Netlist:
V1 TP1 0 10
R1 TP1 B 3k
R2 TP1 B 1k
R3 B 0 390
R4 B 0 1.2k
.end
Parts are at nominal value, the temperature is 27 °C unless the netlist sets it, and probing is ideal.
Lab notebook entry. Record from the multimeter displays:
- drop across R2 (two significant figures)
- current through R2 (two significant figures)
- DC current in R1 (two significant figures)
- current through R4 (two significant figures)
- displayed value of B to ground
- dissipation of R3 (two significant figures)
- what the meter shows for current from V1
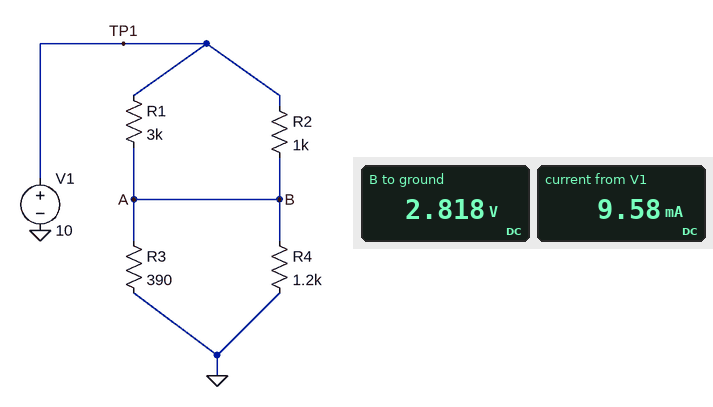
7.2 V
7.2 mA
2.4 mA
2.3 mA
2.818 V
20 mW
9.58 mA
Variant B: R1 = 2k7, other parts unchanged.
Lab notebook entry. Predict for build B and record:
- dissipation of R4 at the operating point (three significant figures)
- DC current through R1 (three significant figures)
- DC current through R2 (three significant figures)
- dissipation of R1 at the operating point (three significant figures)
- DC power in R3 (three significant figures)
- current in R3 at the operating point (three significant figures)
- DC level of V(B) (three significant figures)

6.88 mW
2.64 mA
7.13 mA
18.8 mW
21.2 mW
7.37 mA
2.87 V
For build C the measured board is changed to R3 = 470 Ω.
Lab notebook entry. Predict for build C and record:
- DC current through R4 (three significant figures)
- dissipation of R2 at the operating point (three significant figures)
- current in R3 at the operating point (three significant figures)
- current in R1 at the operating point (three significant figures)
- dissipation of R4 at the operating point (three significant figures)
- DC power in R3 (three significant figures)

2.59 mA
47.5 mW
6.61 mA
2.30 mA
8.03 mW
20.5 mW
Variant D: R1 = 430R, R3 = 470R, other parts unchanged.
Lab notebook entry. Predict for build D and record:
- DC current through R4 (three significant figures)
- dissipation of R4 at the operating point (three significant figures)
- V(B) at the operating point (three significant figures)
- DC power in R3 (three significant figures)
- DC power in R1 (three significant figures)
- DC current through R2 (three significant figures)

4.41 mA
23.3 mW
5.29 V
59.5 mW
51.6 mW
4.71 mA
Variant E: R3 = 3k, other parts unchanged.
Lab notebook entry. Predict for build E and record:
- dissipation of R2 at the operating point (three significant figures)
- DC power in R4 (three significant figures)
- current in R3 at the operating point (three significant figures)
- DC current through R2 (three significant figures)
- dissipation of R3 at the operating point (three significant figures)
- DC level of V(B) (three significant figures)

21.8 mW
23.7 mW
1.78 mA
4.67 mA
9.48 mW
5.33 V
